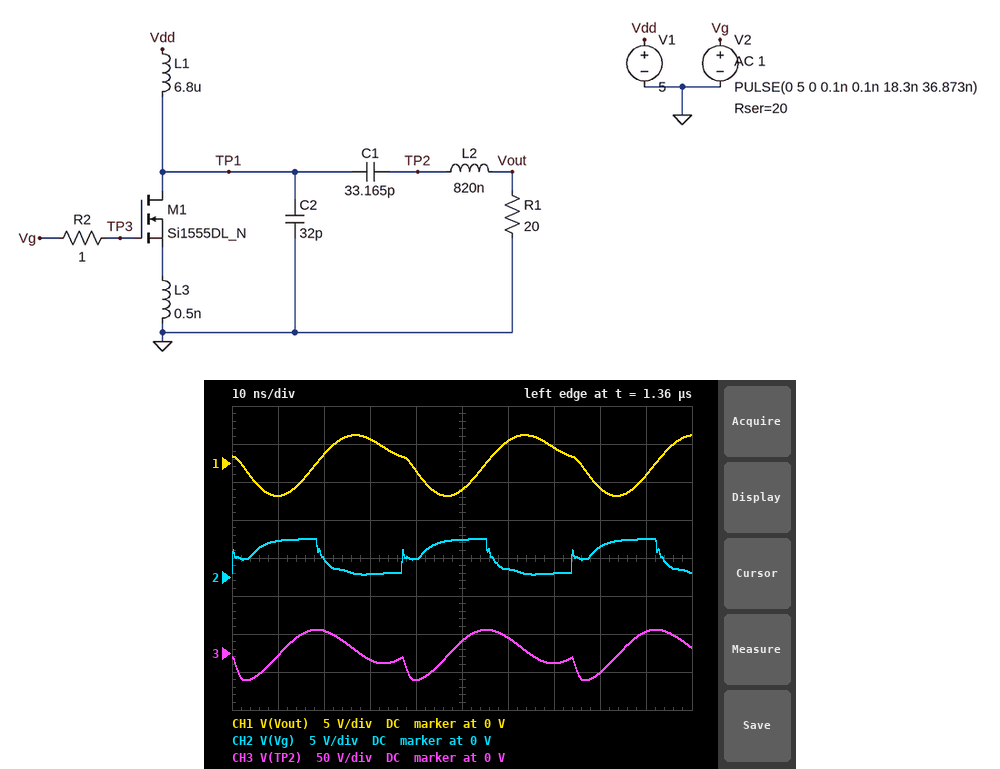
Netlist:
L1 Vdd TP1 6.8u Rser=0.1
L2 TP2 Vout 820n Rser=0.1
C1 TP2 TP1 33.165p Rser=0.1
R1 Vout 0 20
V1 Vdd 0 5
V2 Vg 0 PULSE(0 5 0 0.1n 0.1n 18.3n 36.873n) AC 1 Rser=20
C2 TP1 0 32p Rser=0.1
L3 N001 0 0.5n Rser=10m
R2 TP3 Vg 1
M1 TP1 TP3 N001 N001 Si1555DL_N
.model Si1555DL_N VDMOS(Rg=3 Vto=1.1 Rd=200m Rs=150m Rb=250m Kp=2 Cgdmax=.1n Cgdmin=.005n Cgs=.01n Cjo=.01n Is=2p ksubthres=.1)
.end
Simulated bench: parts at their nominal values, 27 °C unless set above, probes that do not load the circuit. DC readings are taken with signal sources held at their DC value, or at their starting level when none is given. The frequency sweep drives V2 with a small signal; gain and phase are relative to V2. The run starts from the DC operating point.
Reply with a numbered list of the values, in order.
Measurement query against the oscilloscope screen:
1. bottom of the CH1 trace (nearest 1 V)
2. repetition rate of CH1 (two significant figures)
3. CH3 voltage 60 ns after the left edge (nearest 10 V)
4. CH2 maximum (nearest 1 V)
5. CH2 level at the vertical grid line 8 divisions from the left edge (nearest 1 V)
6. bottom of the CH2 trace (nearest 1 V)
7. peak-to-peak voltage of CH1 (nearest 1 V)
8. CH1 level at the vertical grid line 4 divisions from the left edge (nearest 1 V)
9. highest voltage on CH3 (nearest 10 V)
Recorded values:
1. -4 V
2. 27 MHz
3. 20 V
4. 5 V
5. 4 V
6. 0 V
7. 8 V
8. -1 V
9. 30 V
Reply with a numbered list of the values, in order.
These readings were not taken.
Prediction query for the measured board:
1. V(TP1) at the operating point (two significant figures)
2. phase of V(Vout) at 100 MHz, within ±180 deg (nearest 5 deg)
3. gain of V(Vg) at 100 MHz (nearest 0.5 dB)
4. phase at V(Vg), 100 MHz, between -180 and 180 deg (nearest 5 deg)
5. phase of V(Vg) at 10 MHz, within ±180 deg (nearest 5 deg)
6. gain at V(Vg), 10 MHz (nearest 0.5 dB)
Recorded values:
1. 5.0 V
2. -105 deg
3. -0.5 dB
4. -15 deg
5. 0 deg
6. 0 dB
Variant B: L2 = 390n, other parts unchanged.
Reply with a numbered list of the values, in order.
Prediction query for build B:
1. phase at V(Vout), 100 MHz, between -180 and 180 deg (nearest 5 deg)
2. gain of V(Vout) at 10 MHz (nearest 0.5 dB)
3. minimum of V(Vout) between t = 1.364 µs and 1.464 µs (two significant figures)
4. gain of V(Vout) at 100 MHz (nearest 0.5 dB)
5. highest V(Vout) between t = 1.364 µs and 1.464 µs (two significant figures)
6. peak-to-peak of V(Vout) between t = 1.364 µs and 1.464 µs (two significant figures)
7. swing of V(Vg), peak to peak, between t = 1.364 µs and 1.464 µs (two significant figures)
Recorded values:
1. -100 deg
2. -38.5 dB
3. -3.9 V
4. -30.5 dB
5. 2.9 V
6. 6.7 V
7. 5.1 V
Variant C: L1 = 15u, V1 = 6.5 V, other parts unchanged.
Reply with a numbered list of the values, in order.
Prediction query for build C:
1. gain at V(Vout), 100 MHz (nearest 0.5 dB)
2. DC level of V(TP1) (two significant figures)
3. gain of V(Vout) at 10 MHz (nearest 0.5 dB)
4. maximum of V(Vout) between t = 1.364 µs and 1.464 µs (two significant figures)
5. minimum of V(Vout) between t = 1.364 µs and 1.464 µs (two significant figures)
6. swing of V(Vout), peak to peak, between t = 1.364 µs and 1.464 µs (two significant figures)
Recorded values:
1. -39.5 dB
2. 6.5 V
3. -42.5 dB
4. 4.2 V
5. -5.0 V
6. 9.2 V
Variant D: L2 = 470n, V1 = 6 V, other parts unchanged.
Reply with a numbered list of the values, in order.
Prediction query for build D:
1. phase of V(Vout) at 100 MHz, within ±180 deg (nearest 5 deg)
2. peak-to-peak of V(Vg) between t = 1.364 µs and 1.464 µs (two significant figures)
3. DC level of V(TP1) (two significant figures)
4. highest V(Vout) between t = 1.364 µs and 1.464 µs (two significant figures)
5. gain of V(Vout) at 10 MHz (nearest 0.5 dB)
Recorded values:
1. -100 deg
2. 4.8 V
3. 6.0 V
4. 3.0 V
5. -39.0 dB
